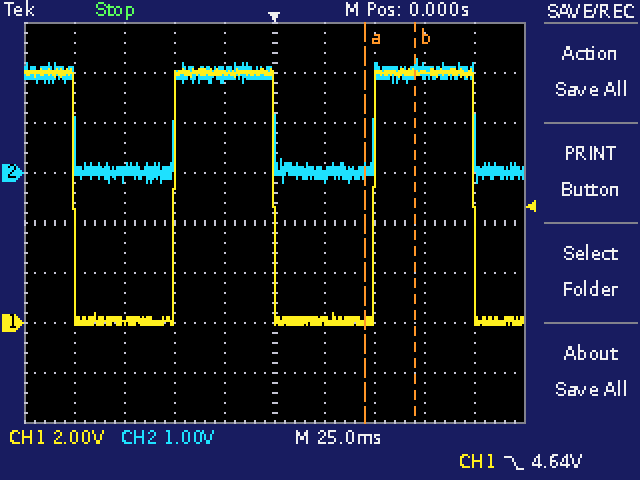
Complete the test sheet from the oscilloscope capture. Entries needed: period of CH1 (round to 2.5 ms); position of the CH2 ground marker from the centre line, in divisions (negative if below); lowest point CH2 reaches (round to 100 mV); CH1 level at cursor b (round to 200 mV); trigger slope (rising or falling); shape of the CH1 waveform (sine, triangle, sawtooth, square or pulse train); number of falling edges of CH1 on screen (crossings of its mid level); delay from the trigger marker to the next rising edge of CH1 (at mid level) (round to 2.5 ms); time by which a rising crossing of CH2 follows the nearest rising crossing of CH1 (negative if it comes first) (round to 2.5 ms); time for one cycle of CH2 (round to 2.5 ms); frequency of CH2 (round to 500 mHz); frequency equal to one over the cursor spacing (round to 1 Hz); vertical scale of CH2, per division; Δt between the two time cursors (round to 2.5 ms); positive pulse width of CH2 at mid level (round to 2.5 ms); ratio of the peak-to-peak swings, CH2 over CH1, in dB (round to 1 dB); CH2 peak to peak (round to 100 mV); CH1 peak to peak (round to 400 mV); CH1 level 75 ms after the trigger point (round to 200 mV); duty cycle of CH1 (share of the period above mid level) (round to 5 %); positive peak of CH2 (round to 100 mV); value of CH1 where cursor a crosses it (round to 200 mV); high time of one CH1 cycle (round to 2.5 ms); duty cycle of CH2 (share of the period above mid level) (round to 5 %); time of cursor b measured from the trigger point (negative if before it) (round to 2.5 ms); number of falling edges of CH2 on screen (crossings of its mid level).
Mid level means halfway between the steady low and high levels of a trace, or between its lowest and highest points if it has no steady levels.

100.0 ms
+1.0 div
-200 mV
10.0 V
falling
square
3
50.0 ms
0.0 ms
100.0 ms
10.0 Hz
40 Hz
1 V
25.0 ms
50.0 ms
-12 dB
2.5 V
10.4 V
10.0 V
50 %
2.3 V
0.0 V
50.0 ms
50 %
+70.0 ms
3
